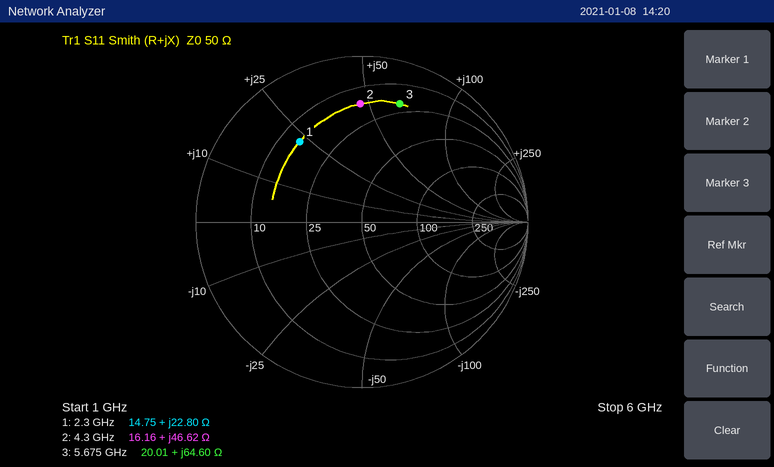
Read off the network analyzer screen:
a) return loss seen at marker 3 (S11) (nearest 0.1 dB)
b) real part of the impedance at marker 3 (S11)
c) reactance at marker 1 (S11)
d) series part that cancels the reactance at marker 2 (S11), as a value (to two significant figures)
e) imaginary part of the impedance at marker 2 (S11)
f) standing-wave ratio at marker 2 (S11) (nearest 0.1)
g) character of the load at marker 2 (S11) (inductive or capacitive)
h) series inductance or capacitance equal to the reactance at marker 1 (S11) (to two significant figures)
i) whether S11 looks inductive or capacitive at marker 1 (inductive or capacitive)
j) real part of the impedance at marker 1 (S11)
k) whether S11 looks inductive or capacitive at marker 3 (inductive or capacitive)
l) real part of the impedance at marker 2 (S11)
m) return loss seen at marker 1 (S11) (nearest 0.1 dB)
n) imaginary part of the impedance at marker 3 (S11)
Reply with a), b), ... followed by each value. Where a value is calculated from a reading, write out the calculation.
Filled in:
a) 2.5 dB
b) 20.01 Ω
c) +22.80 Ω
d) C = 1/(2π × 4.3 GHz × 46.62 Ω) ≈ 794 fF, so 790 fF to two significant figures
e) +46.62 Ω
f) 5.9
g) inductive
h) L = 22.8 Ω/(2π × 2.3 GHz) ≈ 1.6 nH
i) inductive
j) 14.75 Ω
k) inductive
l) 16.16 Ω
m) 4.3 dB
n) +64.60 Ω
